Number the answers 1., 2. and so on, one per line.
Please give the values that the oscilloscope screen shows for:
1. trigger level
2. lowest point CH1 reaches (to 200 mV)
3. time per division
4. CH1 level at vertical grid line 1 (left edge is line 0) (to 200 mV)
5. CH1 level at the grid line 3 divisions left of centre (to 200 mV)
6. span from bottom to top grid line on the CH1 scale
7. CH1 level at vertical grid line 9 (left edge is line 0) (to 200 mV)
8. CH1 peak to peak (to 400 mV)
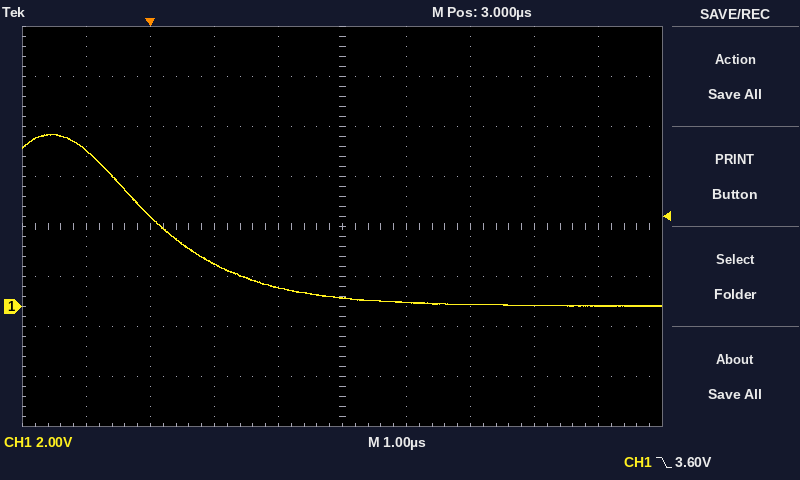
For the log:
1. 3.60 V
2. 0.0 V
3. 1 µs
4. 6.2 V
5. 3.6 V
6. 16 V
7. 0.0 V
8. 6.8 V
